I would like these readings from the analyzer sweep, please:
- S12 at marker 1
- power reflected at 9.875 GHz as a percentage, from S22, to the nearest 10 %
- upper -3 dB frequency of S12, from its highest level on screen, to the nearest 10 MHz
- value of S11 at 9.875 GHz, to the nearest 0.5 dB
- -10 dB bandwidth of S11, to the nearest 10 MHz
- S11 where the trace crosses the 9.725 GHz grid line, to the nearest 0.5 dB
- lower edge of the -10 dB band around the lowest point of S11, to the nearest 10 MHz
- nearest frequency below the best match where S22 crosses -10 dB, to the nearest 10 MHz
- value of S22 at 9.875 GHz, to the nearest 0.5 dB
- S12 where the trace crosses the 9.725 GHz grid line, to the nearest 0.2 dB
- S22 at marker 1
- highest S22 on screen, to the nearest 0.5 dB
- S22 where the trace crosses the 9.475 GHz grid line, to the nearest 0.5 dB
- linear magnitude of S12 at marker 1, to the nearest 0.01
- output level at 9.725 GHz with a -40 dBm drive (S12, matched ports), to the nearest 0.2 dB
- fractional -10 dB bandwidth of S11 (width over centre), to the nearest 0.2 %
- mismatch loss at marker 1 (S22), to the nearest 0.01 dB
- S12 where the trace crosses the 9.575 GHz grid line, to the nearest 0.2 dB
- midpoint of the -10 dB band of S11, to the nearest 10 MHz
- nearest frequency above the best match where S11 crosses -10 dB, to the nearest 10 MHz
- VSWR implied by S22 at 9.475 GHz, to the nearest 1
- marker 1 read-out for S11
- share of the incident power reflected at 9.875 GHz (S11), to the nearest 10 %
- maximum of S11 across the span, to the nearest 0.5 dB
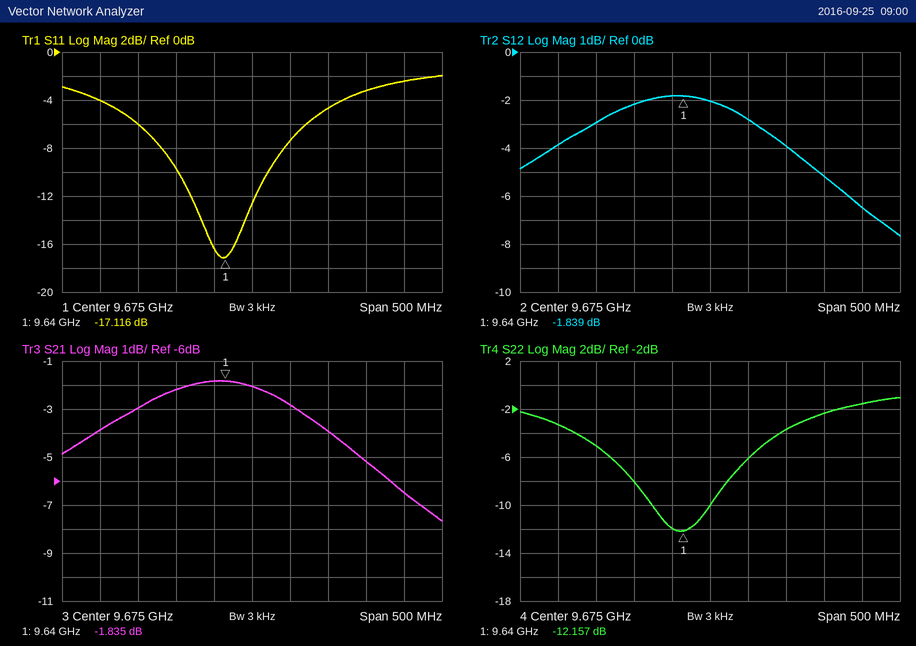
-1.839 dB
70 %
9.81 GHz
-2.5 dB
120 MHz
-7.5 dB
9.58 GHz
9.60 GHz
-1.5 dB
-2.8 dB
-12.157 dB
-1.0 dB
-3.5 dB
0.81
-42.8 dBm
1.2 %
0.27 dB
-2.2 dB
9.64 GHz
9.70 GHz
5
-17.116 dB
60 %
-2.0 dB
